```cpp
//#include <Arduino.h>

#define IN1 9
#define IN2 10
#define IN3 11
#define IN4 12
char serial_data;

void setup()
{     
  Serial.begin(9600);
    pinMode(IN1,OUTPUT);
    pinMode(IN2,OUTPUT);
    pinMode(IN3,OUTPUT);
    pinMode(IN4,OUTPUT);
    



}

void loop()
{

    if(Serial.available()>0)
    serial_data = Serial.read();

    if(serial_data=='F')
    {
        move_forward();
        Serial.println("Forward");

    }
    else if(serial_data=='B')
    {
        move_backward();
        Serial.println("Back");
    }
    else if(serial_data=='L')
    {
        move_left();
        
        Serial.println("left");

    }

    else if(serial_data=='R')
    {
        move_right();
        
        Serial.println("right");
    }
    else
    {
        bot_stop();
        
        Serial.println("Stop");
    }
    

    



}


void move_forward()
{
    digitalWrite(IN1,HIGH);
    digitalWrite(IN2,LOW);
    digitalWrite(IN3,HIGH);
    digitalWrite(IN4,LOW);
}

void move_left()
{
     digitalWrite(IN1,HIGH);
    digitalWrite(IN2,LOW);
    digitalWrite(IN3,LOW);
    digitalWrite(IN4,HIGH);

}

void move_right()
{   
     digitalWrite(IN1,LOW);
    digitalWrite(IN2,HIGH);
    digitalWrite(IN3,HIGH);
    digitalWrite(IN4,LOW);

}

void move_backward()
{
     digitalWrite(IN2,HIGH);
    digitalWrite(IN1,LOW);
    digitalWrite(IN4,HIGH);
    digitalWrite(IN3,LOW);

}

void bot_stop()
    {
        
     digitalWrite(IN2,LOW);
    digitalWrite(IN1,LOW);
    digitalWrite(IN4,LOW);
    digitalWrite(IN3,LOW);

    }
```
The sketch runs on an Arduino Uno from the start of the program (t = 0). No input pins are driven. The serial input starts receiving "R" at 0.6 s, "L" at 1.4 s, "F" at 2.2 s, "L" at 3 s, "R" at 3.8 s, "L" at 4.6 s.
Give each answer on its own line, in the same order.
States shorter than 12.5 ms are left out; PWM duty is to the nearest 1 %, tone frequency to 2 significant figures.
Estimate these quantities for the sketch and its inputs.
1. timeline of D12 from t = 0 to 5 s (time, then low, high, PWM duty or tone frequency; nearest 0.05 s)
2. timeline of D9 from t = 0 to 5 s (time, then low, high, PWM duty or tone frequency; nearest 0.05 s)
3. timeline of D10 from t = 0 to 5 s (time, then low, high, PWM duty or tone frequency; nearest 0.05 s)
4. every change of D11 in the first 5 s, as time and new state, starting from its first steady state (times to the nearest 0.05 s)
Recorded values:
0 s low; 1.4 s high; 2.2 s low; 3 s high; 3.8 s low; 4.6 s high
0 s low; 1.4 s high; 3.8 s low; 4.6 s high
0 s low; 0.6 s high; 1.4 s low; 3.8 s high; 4.6 s low
0 s low; 0.6 s high; 1.4 s low; 2.2 s high; 3 s low; 3.8 s high; 4.6 s low
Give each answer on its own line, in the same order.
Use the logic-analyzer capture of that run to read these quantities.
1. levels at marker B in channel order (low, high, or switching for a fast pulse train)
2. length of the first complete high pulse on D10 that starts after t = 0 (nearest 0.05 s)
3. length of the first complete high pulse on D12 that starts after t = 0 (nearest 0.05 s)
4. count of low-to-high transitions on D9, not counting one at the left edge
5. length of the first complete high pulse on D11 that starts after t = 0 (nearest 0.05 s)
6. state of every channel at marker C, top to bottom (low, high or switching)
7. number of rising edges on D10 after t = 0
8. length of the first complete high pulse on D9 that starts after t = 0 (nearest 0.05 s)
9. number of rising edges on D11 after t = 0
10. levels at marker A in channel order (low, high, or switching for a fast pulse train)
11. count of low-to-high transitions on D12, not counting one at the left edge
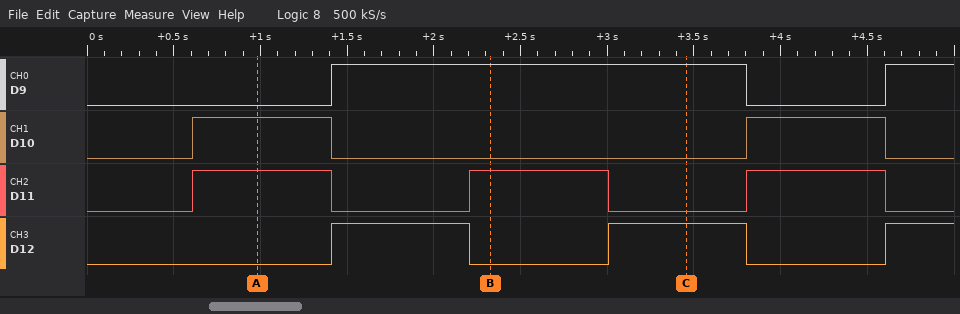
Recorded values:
D9 high, D10 low, D11 high, D12 low
0.80 s
0.80 s
2
0.80 s
D9 high, D10 low, D11 low, D12 high
2
2.40 s
3
D9 low, D10 high, D11 high, D12 low
3
